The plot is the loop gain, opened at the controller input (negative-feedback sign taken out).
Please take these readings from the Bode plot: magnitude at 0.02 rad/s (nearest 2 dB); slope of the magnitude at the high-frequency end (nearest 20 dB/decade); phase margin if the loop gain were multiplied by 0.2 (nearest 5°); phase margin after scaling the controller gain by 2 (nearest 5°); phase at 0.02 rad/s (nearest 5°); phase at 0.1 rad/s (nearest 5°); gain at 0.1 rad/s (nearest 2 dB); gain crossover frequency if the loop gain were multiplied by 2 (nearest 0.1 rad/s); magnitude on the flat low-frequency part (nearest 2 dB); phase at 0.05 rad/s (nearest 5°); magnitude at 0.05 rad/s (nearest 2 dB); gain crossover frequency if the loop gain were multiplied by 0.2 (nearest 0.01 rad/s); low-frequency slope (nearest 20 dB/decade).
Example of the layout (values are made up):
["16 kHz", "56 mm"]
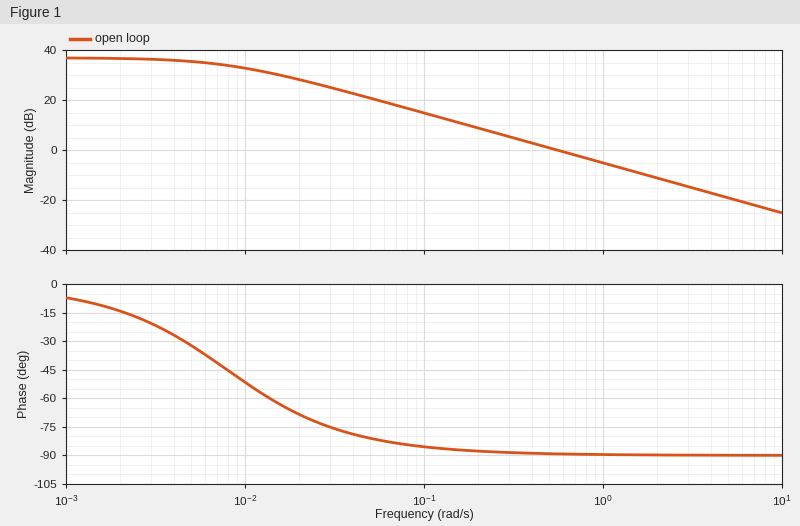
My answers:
["28 dB", "-20 dB/decade", "95°", "90°", "-70°", "-85°", "14 dB", "1.1 rad/s", "36 dB", "-80°", "20 dB", "0.11 rad/s", "0 dB/decade"]
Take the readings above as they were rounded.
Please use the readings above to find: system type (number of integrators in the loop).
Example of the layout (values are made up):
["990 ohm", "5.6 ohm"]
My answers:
["0"]
